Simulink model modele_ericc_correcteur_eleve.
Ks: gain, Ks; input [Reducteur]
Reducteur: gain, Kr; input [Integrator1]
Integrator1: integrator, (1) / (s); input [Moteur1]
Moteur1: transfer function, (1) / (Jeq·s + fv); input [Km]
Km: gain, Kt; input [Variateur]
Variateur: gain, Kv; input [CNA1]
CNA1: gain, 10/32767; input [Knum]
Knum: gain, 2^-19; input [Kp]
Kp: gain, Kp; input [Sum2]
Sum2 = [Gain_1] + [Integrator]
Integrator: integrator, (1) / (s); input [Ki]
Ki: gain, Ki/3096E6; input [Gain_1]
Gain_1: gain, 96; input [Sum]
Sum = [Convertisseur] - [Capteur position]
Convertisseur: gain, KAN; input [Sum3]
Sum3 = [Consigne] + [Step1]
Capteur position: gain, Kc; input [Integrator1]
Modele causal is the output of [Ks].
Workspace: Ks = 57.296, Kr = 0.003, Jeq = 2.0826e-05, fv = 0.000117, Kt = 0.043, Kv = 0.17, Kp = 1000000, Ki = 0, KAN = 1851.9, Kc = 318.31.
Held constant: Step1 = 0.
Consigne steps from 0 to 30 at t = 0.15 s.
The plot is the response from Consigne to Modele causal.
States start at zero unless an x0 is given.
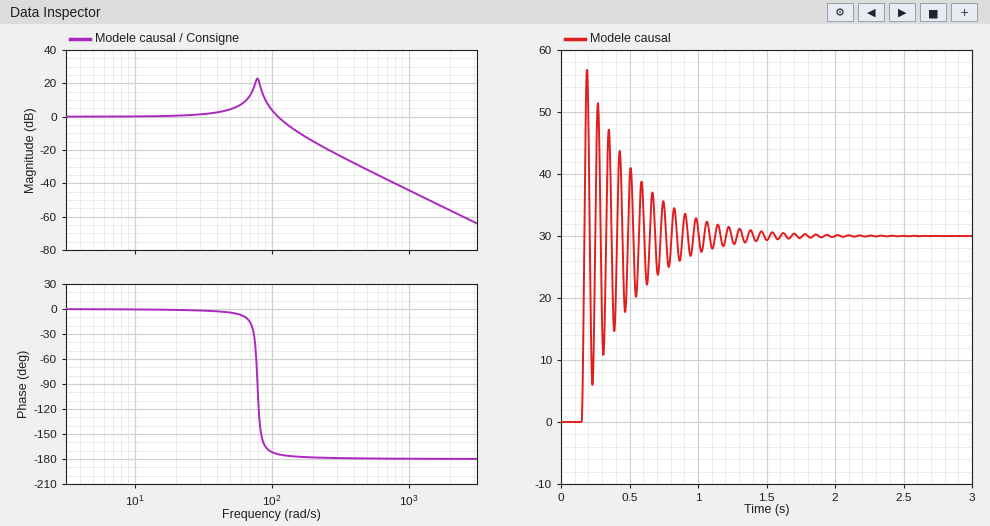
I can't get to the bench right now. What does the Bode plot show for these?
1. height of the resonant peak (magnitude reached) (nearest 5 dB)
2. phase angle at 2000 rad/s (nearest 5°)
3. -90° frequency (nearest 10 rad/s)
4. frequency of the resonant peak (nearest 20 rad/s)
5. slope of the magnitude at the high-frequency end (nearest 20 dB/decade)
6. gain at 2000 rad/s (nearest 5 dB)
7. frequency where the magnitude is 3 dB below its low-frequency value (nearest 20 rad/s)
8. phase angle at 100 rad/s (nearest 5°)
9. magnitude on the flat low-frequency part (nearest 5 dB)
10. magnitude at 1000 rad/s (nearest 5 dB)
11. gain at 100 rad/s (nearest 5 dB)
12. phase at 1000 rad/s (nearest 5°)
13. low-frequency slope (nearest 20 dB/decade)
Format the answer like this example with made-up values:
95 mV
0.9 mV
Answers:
25 dB
-180°
80 rad/s
80 rad/s
-40 dB/decade
-55 dB
120 rad/s
-170°
0 dB
-45 dB
5 dB
-180°
0 dB/decade
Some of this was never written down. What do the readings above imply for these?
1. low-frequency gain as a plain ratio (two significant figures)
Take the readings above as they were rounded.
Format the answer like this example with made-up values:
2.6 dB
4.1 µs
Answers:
1.0
